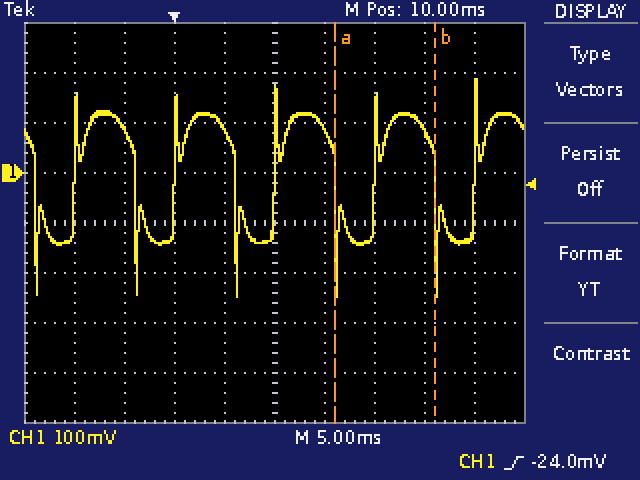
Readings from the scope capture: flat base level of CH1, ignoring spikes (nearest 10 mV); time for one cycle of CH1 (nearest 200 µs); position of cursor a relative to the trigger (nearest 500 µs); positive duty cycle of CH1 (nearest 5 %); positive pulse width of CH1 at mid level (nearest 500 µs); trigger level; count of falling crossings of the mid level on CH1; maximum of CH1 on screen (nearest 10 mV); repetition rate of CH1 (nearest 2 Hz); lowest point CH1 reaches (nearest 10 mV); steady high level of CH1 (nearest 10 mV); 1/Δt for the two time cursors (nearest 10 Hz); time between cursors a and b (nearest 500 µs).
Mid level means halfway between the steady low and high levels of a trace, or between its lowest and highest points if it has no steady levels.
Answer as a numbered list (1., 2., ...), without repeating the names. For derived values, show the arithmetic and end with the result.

1. -140 mV
2. 10.0 ms
3. +16.0 ms
4. 6.0 ms / 10.0 ms ≈ 60 %
5. 6.0 ms
6. -24.0 mV
7. 5
8. 190 mV
9. 1 / 10.0 ms ≈ 100 Hz
10. -250 mV
11. 120 mV
12. 1 / 10.0 ms ≈ 100 Hz
13. 10.0 ms
